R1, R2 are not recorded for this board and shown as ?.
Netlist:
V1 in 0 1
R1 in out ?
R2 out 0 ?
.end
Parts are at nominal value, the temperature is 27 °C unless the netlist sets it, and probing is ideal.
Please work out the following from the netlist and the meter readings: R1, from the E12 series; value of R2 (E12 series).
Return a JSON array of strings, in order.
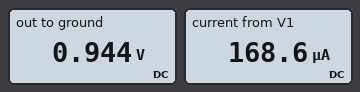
["330 Ω", "5.6 kΩ"]
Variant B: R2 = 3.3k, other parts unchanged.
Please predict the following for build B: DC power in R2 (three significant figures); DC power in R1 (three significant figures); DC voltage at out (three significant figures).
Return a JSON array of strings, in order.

["250 µW", "25.0 µW", "909 mV"]
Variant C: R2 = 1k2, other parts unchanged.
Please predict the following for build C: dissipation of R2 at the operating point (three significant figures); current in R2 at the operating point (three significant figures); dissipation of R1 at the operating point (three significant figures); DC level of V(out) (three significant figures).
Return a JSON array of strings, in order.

["513 µW", "654 µA", "141 µW", "784 mV"]
